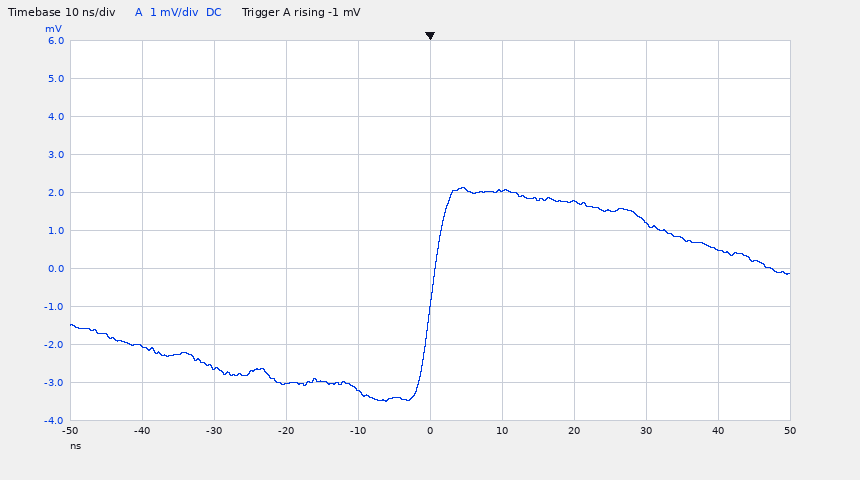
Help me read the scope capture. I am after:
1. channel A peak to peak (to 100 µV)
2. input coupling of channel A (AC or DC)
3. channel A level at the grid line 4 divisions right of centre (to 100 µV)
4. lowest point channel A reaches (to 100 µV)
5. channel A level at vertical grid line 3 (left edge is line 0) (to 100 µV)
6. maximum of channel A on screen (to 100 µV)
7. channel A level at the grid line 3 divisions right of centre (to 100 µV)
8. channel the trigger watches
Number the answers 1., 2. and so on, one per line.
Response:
1. 5.6 mV
2. DC
3. 500 µV
4. -3.5 mV
5. -3.0 mV
6. 2.1 mV
7. 1.2 mV
8. channel A
